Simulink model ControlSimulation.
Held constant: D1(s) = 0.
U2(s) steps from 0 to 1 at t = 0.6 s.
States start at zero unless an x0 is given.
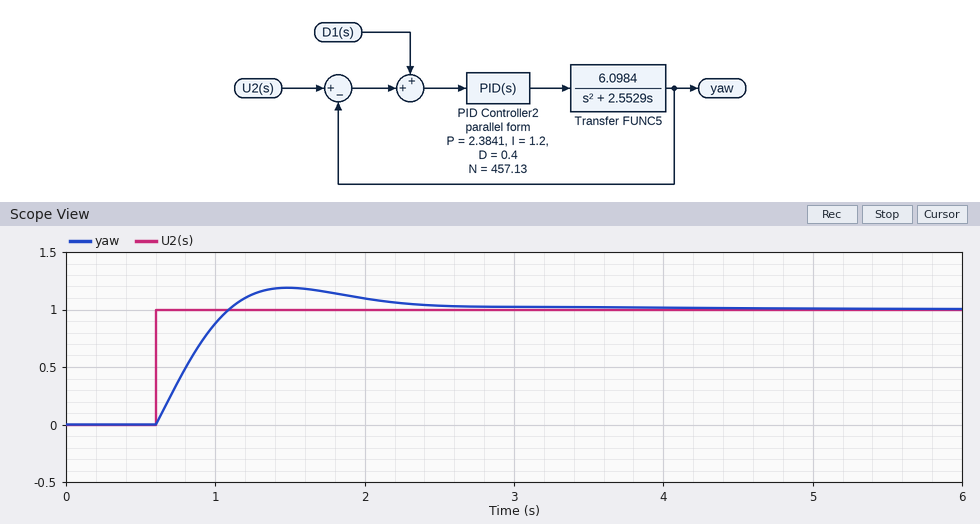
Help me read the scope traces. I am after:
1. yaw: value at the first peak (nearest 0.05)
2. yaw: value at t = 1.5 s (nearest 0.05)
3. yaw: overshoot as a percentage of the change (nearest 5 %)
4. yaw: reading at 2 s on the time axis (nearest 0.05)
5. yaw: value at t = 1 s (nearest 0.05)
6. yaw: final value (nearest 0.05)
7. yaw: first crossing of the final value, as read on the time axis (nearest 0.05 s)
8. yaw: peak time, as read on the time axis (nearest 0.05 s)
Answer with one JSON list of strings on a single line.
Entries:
["1.20", "1.20", "20 %", "1.10", "0.90", "1.00", "1.10 s", "1.50 s"]
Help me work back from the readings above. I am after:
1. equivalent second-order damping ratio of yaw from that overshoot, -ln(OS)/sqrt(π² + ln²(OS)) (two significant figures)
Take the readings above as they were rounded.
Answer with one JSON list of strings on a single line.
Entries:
["0.46"]
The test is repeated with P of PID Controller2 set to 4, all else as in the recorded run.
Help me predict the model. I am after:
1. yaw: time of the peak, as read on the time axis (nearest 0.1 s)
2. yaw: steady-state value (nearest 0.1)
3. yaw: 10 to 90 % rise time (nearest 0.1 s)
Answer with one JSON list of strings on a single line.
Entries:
["1.2 s", "1.0", "0.3 s"]
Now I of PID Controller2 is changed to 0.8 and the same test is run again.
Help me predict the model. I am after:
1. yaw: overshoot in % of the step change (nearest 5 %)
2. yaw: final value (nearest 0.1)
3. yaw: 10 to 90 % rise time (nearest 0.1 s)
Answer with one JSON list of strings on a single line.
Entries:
["15 %", "1.0", "0.4 s"]
